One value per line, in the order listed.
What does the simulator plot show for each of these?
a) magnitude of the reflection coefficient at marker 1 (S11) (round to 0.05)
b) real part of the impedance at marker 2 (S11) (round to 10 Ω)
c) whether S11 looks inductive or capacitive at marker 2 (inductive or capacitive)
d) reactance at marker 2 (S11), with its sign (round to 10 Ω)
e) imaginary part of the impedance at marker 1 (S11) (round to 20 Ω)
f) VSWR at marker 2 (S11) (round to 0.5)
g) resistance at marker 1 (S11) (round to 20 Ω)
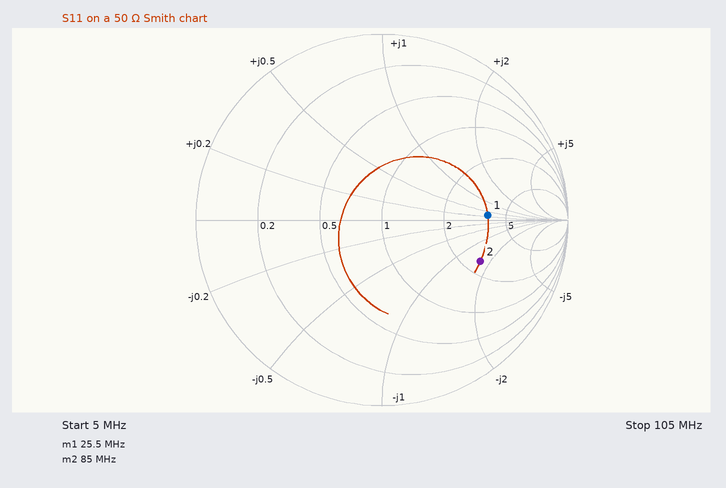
0.55
120 Ω
capacitive
-80 Ω
+20 Ω
3.5
180 Ω
